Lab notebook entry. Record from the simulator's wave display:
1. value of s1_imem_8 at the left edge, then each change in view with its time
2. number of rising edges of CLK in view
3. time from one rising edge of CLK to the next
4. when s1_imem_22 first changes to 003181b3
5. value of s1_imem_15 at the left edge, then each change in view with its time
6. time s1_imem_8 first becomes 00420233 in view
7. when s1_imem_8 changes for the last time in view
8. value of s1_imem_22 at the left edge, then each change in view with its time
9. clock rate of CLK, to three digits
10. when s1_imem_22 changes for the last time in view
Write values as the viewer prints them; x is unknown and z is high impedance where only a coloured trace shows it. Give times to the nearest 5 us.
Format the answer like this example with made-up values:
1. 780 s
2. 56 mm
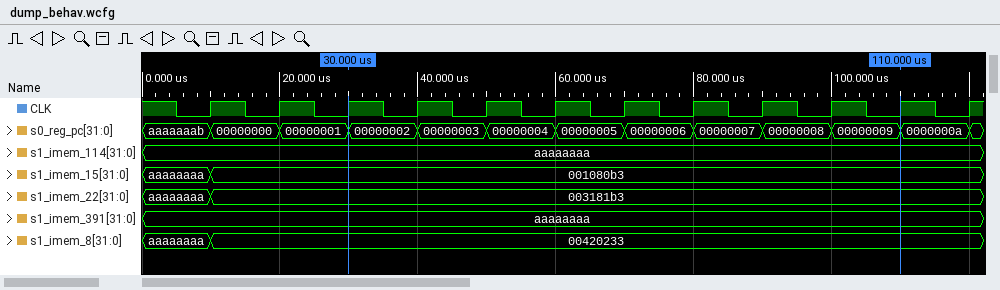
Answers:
1. aaaaaaaa, 00420233 at 10 us
2. 12
3. 10 us
4. 10 us
5. aaaaaaaa, 001080b3 at 10 us
6. 10 us
7. 10 us
8. aaaaaaaa, 003181b3 at 10 us
9. 100 kHz
10. 10 us
